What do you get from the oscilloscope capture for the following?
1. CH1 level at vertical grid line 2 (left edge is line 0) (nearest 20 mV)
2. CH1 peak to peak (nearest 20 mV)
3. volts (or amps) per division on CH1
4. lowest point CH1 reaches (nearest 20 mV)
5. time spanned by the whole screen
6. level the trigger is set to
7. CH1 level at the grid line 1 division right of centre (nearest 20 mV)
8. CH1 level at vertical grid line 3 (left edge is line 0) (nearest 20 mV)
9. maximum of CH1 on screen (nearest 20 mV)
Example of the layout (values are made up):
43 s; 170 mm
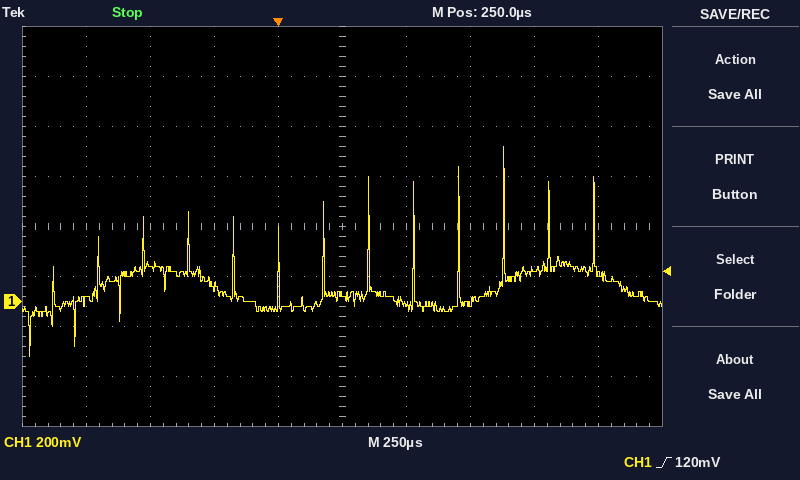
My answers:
140 mV; 840 mV; 200 mV; -220 mV; 2.5 ms; 120 mV; -20 mV; 60 mV; 620 mV
